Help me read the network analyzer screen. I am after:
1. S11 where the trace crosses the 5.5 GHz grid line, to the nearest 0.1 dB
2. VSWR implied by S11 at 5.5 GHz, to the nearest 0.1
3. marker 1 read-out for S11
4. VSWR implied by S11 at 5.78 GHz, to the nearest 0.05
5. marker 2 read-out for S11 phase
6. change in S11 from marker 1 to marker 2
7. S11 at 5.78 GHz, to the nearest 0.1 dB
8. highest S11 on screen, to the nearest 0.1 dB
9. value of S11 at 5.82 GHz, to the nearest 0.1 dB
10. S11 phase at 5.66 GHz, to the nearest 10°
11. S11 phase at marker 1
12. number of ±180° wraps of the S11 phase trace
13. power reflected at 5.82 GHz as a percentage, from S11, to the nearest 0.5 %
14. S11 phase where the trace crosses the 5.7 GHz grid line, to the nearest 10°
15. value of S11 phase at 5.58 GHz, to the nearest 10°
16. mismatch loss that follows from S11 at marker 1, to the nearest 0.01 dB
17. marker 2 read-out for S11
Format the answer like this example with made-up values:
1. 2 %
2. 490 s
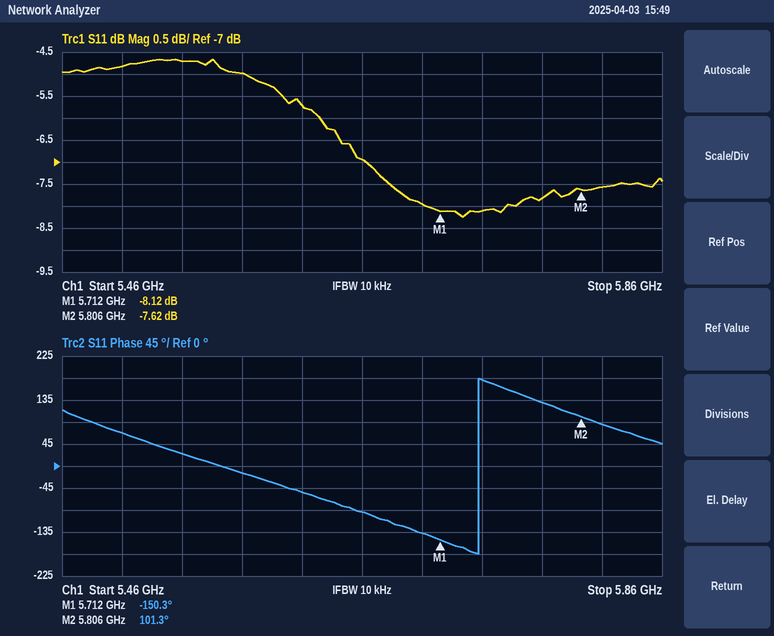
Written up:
1. -4.8 dB
2. 3.7
3. -8.12 dB
4. 2.35
5. 101.3°
6. 0.50 dB
7. -7.8 dB
8. -4.7 dB
9. -7.6 dB
10. -90°
11. -150.3°
12. 1
13. 17.5 %
14. -140°
15. -10°
16. 0.73 dB
17. -7.62 dB
